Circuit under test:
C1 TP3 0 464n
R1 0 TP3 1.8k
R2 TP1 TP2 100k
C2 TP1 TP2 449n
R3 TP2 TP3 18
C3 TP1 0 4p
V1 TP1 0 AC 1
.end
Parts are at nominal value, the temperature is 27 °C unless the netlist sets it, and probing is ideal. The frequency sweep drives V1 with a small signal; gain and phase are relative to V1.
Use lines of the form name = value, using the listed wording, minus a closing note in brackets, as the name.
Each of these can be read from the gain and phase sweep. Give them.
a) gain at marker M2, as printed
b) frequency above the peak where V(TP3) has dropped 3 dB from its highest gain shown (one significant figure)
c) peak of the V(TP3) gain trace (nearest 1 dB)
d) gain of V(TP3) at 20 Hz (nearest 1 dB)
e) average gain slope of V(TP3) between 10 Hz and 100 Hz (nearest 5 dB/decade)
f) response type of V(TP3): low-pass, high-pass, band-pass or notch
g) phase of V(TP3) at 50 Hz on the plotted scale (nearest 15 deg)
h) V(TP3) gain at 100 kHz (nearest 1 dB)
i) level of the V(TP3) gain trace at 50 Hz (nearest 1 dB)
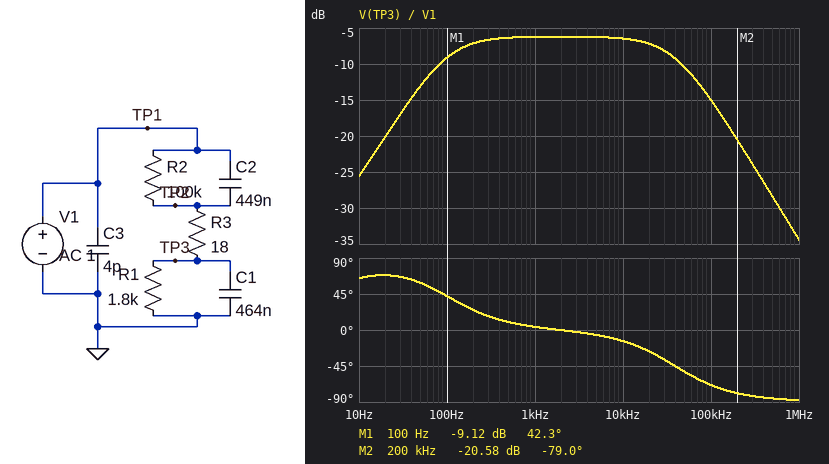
gain at marker M2, as printed = -20.58 dB
frequency above the peak where V(TP3) has dropped 3 dB from its highest gain shown = 40 kHz
peak of the V(TP3) gain trace = -6 dB
gain of V(TP3) at 20 Hz = -20 dB
average gain slope of V(TP3) between 10 Hz and 100 Hz = 15 dB/decade
response type of V(TP3): low-pass, high-pass, band-pass or notch = band-pass
phase of V(TP3) at 50 Hz on the plotted scale = 60 deg
V(TP3) gain at 100 kHz = -15 dB
level of the V(TP3) gain trace at 50 Hz = -13 dB
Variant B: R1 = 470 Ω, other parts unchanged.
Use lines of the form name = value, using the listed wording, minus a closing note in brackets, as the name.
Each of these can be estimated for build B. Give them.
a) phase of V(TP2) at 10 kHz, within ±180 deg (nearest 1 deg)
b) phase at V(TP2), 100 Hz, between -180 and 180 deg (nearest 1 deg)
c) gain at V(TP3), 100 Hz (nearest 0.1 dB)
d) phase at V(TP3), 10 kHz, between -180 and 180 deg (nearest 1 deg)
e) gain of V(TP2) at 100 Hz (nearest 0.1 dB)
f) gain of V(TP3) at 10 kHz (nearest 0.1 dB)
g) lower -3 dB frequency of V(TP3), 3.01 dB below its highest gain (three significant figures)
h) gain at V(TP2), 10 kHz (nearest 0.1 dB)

phase of V(TP2) at 10 kHz, within ±180 deg = 15 deg
phase at V(TP2), 100 Hz, between -180 and 180 deg = 73 deg
gain at V(TP3), 100 Hz = -17.9 dB
phase at V(TP3), 10 kHz, between -180 and 180 deg = -12 deg
gain of V(TP2) at 100 Hz = -17.6 dB
gain of V(TP3) at 10 kHz = -6.5 dB
lower -3 dB frequency of V(TP3), 3.01 dB below its highest gain = 362 Hz
gain at V(TP2), 10 kHz = -5.2 dB
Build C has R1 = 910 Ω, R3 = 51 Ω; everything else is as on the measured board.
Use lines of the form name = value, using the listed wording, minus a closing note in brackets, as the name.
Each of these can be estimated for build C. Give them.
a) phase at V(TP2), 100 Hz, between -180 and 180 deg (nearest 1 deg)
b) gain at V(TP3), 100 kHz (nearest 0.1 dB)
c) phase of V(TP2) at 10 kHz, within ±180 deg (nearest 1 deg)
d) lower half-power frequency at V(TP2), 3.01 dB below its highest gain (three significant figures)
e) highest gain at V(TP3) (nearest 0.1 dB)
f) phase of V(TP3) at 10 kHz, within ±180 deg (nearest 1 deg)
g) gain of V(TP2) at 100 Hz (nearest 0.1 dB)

phase at V(TP2), 100 Hz, between -180 and 180 deg = 61 deg
gain at V(TP3), 100 kHz = -23.5 dB
phase of V(TP2) at 10 kHz, within ±180 deg = 20 deg
lower half-power frequency at V(TP2), 3.01 dB below its highest gain = 9.56 kHz
highest gain at V(TP3) = -6.4 dB
phase of V(TP3) at 10 kHz, within ±180 deg = -35 deg
gain of V(TP2) at 100 Hz = -12.5 dB
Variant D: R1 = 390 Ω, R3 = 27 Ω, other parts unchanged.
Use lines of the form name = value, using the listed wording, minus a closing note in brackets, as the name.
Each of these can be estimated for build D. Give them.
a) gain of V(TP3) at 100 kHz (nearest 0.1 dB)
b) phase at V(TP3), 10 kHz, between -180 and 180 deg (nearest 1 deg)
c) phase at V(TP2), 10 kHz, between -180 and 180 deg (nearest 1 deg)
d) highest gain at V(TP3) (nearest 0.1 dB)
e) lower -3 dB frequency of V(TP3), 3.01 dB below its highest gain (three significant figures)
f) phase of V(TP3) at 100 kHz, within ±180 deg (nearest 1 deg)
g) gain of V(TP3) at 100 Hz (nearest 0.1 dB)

gain of V(TP3) at 100 kHz = -18.2 dB
phase at V(TP3), 10 kHz, between -180 and 180 deg = -18 deg
phase at V(TP2), 10 kHz, between -180 and 180 deg = 18 deg
highest gain at V(TP3) = -6.5 dB
lower -3 dB frequency of V(TP3), 3.01 dB below its highest gain = 427 Hz
phase of V(TP3) at 100 kHz, within ±180 deg = -75 deg
gain of V(TP3) at 100 Hz = -19.4 dB
